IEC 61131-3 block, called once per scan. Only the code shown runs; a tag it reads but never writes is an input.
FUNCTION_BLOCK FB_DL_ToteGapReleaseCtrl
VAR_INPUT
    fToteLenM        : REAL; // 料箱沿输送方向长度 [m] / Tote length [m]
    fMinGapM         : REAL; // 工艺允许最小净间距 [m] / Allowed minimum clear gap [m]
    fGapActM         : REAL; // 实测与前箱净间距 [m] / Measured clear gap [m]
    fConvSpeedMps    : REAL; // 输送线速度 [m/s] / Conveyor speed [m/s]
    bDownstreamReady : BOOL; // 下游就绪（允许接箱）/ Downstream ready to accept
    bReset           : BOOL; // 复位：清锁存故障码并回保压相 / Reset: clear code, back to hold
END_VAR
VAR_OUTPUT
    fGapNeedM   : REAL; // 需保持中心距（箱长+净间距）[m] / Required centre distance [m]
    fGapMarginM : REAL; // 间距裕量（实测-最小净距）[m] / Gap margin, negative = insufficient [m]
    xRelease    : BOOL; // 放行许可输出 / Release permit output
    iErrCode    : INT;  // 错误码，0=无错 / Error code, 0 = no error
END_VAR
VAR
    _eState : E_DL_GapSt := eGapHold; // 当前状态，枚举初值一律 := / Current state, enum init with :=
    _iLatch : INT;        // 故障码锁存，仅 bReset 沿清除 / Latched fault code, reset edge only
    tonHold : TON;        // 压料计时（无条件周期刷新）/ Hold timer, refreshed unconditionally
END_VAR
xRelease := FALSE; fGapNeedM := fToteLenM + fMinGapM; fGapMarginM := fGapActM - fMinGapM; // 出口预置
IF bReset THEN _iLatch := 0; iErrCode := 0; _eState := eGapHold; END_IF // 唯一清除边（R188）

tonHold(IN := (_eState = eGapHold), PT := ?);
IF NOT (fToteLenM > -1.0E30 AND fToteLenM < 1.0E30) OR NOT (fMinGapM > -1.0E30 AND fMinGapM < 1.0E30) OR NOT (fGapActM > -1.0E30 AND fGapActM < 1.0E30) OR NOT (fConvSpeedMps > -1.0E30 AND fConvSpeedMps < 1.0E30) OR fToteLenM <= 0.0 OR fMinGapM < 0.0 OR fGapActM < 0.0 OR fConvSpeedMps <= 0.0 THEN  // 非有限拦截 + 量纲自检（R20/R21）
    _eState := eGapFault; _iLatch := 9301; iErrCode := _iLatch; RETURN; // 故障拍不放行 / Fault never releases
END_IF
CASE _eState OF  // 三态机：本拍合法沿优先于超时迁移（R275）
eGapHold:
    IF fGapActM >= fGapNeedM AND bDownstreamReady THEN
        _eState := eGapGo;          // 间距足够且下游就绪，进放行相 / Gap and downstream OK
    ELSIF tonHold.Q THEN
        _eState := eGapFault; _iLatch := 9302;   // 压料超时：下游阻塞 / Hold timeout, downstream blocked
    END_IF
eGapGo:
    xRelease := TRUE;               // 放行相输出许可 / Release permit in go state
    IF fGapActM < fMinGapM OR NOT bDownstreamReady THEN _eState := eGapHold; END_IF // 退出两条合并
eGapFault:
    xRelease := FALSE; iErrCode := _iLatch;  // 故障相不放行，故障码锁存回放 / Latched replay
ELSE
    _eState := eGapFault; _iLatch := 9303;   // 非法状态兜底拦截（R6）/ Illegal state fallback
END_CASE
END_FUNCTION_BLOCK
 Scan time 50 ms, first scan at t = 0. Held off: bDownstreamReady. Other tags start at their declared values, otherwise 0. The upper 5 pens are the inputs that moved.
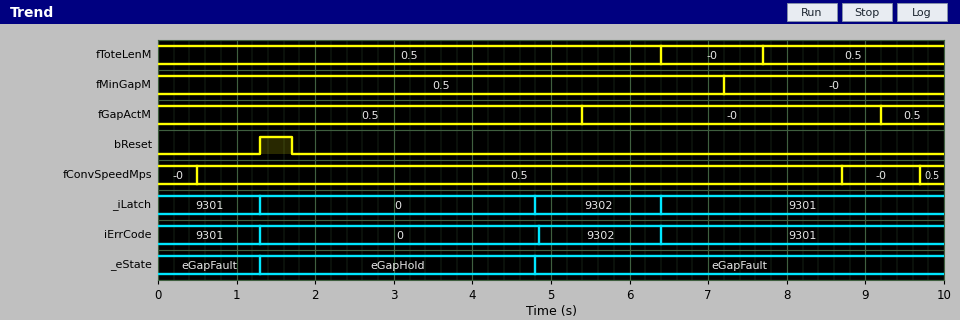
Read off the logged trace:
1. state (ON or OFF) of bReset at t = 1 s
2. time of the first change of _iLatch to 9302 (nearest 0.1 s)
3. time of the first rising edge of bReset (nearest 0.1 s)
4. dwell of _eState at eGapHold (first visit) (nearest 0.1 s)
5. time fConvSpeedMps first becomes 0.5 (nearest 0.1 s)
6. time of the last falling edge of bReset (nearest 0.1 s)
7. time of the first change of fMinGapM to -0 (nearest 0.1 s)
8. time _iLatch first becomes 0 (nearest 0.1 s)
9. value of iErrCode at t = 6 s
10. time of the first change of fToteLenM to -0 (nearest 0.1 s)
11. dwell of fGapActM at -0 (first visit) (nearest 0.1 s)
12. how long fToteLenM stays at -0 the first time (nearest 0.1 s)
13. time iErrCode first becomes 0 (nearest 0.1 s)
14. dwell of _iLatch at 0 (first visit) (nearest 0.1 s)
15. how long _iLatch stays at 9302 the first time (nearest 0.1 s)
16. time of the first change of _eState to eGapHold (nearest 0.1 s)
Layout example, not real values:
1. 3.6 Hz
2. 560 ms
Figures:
1. OFF
2. 4.8 s
3. 1.3 s
4. 3.5 s
5. 0.5 s
6. 1.7 s
7. 7.2 s
8. 1.3 s
9. 9302
10. 6.4 s
11. 3.8 s
12. 1.3 s
13. 1.3 s
14. 3.5 s
15. 1.6 s
16. 1.3 s
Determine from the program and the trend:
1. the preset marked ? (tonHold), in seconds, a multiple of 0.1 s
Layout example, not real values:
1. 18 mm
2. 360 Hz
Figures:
1. 3.5 s
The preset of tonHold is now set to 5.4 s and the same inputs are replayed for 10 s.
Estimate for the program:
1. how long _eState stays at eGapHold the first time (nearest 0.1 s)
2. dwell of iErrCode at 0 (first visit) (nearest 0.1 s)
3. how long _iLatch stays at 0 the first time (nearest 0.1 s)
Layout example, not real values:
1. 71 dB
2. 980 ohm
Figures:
1. 5.1 s
2. 5.1 s
3. 5.1 s
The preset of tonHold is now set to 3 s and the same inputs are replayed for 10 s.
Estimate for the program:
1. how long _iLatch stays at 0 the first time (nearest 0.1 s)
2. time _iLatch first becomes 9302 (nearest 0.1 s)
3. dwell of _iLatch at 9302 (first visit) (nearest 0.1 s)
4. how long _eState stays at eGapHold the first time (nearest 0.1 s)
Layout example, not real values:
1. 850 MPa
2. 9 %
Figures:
1. 3.0 s
2. 4.3 s
3. 2.1 s
4. 3.0 s
